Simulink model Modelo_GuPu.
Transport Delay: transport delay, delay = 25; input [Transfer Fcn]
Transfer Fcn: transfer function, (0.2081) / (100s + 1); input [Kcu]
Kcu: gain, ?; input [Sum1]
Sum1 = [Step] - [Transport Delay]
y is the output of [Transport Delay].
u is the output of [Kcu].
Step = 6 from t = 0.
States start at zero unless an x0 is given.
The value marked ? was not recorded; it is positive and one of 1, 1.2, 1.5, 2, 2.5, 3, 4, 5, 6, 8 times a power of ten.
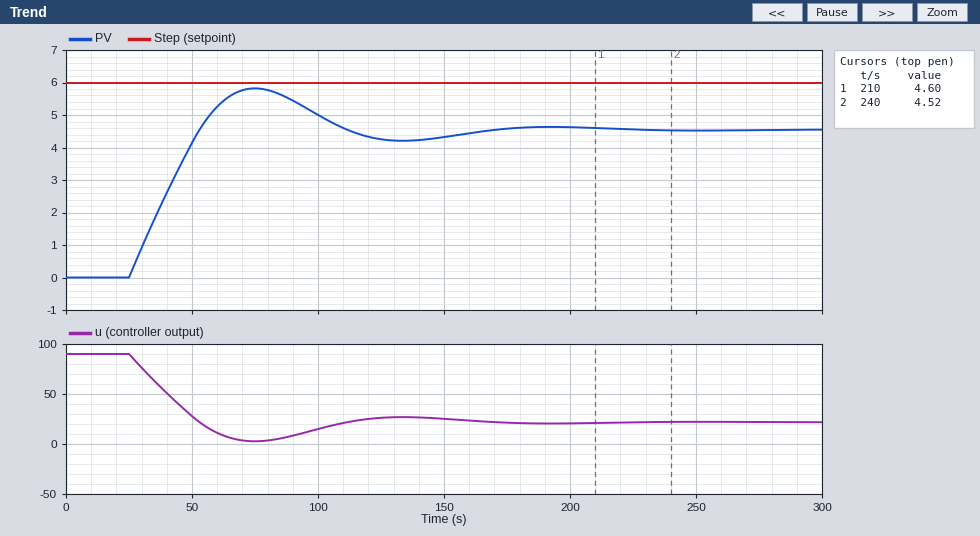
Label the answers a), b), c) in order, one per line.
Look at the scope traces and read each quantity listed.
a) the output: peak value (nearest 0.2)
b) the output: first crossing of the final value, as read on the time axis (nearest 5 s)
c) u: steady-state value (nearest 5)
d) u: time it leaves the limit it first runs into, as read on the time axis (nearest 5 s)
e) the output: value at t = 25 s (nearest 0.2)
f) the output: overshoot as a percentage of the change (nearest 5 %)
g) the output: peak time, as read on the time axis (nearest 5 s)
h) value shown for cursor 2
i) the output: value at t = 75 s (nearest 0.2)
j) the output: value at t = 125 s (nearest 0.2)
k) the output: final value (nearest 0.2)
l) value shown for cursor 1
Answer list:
a) 5.8
b) 55 s
c) 20
d) 25 s
e) 0.0
f) 30 %
g) 75 s
h) 4.52
i) 5.8
j) 4.2
k) 4.6
l) 4.60
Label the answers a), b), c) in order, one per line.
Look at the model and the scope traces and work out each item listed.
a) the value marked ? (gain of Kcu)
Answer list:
a) 15
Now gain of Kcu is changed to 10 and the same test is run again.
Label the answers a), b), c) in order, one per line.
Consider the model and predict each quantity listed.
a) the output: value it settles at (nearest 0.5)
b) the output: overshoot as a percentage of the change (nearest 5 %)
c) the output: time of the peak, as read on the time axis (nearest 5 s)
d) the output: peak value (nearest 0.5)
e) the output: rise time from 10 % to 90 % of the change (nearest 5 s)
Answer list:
a) 4.0
b) 10 %
c) 90 s
d) 4.5
e) 35 s
